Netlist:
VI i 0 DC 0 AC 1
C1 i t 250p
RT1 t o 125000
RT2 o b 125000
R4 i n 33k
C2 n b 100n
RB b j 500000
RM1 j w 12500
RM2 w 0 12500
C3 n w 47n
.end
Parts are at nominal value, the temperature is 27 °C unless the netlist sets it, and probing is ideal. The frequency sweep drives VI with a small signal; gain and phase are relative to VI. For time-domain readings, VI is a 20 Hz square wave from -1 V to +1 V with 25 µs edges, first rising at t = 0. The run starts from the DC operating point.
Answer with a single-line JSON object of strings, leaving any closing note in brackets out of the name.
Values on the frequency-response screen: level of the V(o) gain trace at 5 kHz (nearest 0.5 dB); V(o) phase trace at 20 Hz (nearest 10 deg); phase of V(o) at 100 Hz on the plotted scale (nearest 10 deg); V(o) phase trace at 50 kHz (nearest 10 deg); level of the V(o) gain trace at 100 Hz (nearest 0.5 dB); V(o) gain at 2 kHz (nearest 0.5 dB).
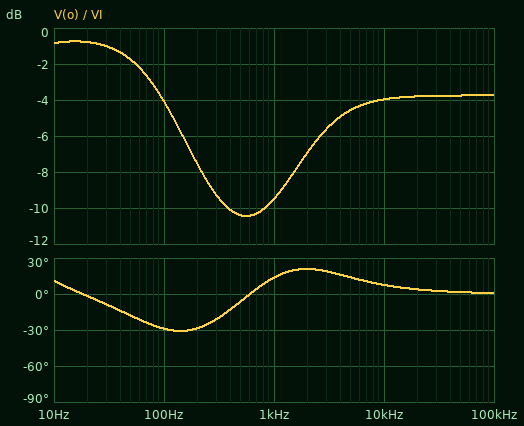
{"level of the V(o) gain trace at 5 kHz": "-4.5 dB", "V(o) phase trace at 20 Hz": "0 deg", "phase of V(o) at 100 Hz on the plotted scale": "-30 deg", "V(o) phase trace at 50 kHz": "0 deg", "level of the V(o) gain trace at 100 Hz": "-4.0 dB", "V(o) gain at 2 kHz": "-7.0 dB"}
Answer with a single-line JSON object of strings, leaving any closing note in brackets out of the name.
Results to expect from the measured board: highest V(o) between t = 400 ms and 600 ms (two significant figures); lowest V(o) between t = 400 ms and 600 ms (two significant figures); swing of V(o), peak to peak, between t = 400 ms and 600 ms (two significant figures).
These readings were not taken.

{"highest V(o) between t = 400 ms and 600 ms": "1.0 V", "lowest V(o) between t = 400 ms and 600 ms": "-1.0 V", "swing of V(o), peak to peak, between t = 400 ms and 600 ms": "2.0 V"}
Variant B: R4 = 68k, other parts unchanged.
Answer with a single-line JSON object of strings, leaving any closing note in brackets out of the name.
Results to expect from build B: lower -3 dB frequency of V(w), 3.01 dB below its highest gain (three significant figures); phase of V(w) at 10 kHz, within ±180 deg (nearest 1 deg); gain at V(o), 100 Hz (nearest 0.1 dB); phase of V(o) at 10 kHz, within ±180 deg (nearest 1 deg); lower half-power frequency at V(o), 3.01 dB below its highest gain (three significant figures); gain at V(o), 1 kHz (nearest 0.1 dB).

{"lower -3 dB frequency of V(w), 3.01 dB below its highest gain": "82.6 Hz", "phase of V(w) at 10 kHz, within ±180 deg": "3 deg", "gain at V(o), 100 Hz": "-7.9 dB", "phase of V(o) at 10 kHz, within ±180 deg": "10 deg", "lower half-power frequency at V(o), 3.01 dB below its highest gain": "2.41 Hz", "gain at V(o), 1 kHz": "-12.1 dB"}
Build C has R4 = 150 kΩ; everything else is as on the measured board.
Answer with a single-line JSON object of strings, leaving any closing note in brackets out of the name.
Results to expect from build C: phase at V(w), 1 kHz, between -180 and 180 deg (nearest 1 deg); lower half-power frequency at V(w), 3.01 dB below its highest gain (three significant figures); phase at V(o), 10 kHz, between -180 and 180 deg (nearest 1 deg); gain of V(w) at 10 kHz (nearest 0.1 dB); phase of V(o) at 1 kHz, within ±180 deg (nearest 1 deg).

{"phase at V(w), 1 kHz, between -180 and 180 deg": "11 deg", "lower half-power frequency at V(w), 3.01 dB below its highest gain": "961 Hz", "phase at V(o), 10 kHz, between -180 and 180 deg": "12 deg", "gain of V(w) at 10 kHz": "-18.7 dB", "phase of V(o) at 1 kHz, within ±180 deg": "45 deg"}
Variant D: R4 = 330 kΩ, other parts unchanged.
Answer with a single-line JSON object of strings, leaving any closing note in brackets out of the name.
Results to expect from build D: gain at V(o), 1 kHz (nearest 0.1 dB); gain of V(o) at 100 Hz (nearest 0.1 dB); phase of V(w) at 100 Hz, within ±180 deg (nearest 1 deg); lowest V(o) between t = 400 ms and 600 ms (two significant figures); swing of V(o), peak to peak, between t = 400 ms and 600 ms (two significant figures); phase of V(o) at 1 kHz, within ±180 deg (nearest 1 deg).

{"gain at V(o), 1 kHz": "-14.0 dB", "gain of V(o) at 100 Hz": "-20.7 dB", "phase of V(w) at 100 Hz, within ±180 deg": "8 deg", "lowest V(o) between t = 400 ms and 600 ms": "-480 mV", "swing of V(o), peak to peak, between t = 400 ms and 600 ms": "960 mV", "phase of V(o) at 1 kHz, within ±180 deg": "56 deg"}
